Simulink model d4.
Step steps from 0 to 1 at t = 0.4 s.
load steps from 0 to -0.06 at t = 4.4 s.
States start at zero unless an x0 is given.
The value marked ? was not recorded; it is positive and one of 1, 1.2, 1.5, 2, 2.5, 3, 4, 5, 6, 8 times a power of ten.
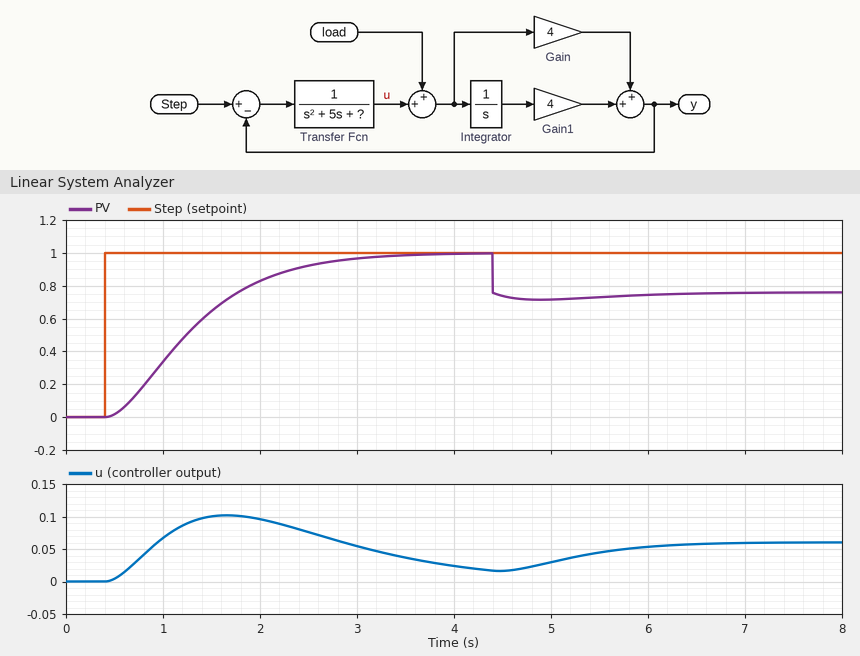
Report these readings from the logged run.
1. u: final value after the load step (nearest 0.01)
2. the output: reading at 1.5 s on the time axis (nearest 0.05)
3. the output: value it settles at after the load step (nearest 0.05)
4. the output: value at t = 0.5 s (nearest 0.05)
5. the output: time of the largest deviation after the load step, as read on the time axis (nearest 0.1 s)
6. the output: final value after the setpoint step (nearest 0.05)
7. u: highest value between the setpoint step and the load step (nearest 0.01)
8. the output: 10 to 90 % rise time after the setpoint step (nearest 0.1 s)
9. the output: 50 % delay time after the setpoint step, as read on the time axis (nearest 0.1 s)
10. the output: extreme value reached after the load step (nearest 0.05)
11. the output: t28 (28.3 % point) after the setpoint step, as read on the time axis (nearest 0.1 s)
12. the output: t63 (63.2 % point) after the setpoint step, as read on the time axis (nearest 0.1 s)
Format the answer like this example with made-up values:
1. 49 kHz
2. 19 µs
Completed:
1. 0.06
2. 0.65
3. 0.75
4. 0.00
5. 4.9 s
6. 1.00
7. 0.10
8. 1.7 s
9. 1.2 s
10. 0.70
11. 0.9 s
12. 1.5 s
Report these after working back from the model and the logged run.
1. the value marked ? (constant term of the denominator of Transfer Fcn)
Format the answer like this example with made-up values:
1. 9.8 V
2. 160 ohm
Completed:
1. 4
